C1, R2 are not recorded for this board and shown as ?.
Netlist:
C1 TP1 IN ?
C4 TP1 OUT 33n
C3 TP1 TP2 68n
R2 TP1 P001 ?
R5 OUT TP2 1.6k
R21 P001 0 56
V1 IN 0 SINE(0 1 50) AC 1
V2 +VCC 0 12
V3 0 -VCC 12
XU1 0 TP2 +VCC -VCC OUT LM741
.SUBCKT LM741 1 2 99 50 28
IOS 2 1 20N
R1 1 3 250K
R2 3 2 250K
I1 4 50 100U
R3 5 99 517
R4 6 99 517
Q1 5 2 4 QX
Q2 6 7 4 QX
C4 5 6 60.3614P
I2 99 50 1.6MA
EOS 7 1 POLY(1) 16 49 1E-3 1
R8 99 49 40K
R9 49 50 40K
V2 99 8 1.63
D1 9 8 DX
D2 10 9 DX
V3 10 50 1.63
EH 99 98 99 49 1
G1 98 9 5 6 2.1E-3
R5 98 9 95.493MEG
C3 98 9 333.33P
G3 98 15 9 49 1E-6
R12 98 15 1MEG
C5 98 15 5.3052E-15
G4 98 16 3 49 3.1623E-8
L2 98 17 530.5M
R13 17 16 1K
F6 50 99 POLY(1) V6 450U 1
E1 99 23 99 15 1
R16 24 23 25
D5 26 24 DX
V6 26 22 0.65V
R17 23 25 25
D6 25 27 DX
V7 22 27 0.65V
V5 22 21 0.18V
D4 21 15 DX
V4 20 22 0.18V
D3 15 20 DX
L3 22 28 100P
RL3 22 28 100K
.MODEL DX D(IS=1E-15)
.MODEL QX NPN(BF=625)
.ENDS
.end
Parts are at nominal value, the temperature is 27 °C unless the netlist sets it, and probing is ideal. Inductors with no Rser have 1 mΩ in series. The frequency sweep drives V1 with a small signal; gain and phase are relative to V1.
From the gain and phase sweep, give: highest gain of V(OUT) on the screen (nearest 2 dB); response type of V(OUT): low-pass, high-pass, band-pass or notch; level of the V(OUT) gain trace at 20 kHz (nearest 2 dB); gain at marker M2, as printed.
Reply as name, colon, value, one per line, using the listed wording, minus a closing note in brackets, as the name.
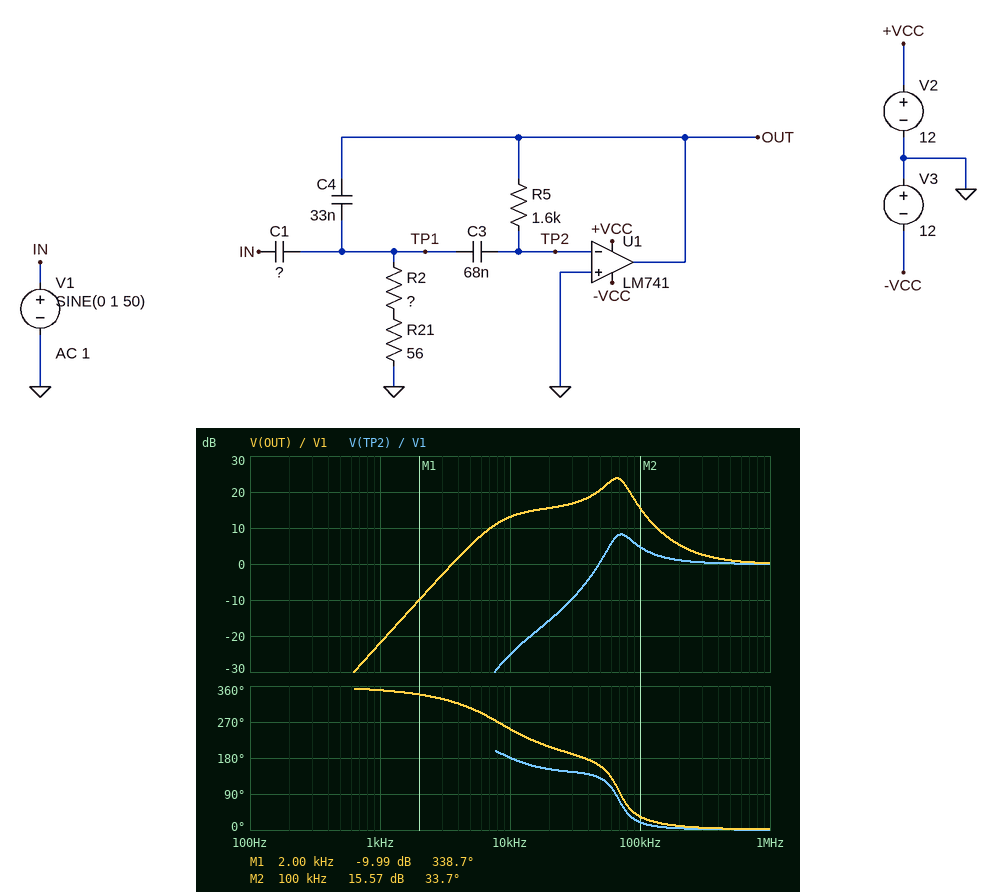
highest gain of V(OUT) on the screen: 24 dB
response type of V(OUT): low-pass, high-pass, band-pass or notch: band-pass
level of the V(OUT) gain trace at 20 kHz: 16 dB
gain at marker M2, as printed: 15.57 dB
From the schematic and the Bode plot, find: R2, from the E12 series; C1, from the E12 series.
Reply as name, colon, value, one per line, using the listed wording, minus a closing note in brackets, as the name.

R2, from the E12 series: 47 Ω
C1, from the E12 series: 180 nF
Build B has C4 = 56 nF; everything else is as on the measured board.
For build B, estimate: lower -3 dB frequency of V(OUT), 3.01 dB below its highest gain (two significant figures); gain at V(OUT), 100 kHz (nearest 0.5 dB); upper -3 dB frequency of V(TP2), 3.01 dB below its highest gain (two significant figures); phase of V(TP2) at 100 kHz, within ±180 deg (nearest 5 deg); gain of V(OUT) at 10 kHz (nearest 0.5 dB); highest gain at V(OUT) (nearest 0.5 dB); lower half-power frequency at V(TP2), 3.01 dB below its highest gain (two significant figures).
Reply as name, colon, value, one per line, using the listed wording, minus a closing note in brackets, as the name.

lower -3 dB frequency of V(OUT), 3.01 dB below its highest gain: 57 kHz
gain at V(OUT), 100 kHz: 13.0 dB
upper -3 dB frequency of V(TP2), 3.01 dB below its highest gain: 87 kHz
phase of V(TP2) at 100 kHz, within ±180 deg: 15 deg
gain of V(OUT) at 10 kHz: 10.5 dB
highest gain at V(OUT): 22.5 dB
lower half-power frequency at V(TP2), 3.01 dB below its highest gain: 62 kHz
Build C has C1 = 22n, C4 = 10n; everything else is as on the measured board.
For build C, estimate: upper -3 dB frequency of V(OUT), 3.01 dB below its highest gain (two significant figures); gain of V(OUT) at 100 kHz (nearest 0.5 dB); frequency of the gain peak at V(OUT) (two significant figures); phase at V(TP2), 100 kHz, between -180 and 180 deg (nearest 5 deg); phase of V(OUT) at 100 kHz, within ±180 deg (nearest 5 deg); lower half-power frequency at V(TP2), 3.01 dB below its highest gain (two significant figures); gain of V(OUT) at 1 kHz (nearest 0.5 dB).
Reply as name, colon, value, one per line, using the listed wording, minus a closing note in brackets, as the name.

upper -3 dB frequency of V(OUT), 3.01 dB below its highest gain: 300 kHz
gain of V(OUT) at 100 kHz: 8.0 dB
frequency of the gain peak at V(OUT): 200 kHz
phase at V(TP2), 100 kHz, between -180 and 180 deg: 115 deg
phase of V(OUT) at 100 kHz, within ±180 deg: 155 deg
lower half-power frequency at V(TP2), 3.01 dB below its highest gain: 170 kHz
gain of V(OUT) at 1 kHz: -40.0 dB
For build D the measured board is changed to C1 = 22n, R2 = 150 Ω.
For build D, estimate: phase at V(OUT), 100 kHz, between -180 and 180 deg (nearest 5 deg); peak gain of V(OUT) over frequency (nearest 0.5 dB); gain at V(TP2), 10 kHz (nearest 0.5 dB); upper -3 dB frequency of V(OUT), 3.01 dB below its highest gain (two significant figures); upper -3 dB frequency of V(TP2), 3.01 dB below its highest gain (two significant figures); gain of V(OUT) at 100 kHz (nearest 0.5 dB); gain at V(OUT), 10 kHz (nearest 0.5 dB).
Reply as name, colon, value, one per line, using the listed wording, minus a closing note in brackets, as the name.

phase at V(OUT), 100 kHz, between -180 and 180 deg: 165 deg
peak gain of V(OUT) over frequency: 12.0 dB
gain at V(TP2), 10 kHz: -40.5 dB
upper -3 dB frequency of V(OUT), 3.01 dB below its highest gain: 250 kHz
upper -3 dB frequency of V(TP2), 3.01 dB below its highest gain: 280 kHz
gain of V(OUT) at 100 kHz: 1.5 dB
gain at V(OUT), 10 kHz: -2.0 dB
